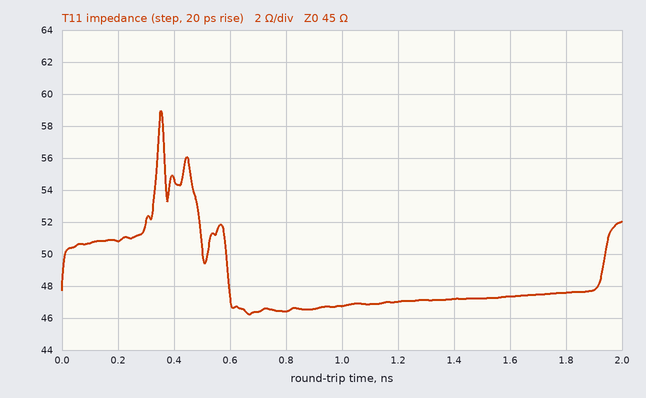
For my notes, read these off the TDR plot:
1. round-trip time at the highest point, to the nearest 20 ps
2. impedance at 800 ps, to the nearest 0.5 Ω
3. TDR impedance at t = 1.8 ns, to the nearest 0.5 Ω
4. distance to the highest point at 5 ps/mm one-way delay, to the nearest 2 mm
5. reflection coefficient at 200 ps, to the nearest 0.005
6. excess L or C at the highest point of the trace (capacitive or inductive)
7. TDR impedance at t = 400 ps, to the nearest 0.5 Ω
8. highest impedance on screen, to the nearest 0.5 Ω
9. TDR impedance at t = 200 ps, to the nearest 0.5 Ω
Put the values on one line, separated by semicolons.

360 ps; 46.5 Ω; 47.5 Ω; 36 mm; +0.060; inductive; 54.5 Ω; 59.0 Ω; 51.0 Ω
